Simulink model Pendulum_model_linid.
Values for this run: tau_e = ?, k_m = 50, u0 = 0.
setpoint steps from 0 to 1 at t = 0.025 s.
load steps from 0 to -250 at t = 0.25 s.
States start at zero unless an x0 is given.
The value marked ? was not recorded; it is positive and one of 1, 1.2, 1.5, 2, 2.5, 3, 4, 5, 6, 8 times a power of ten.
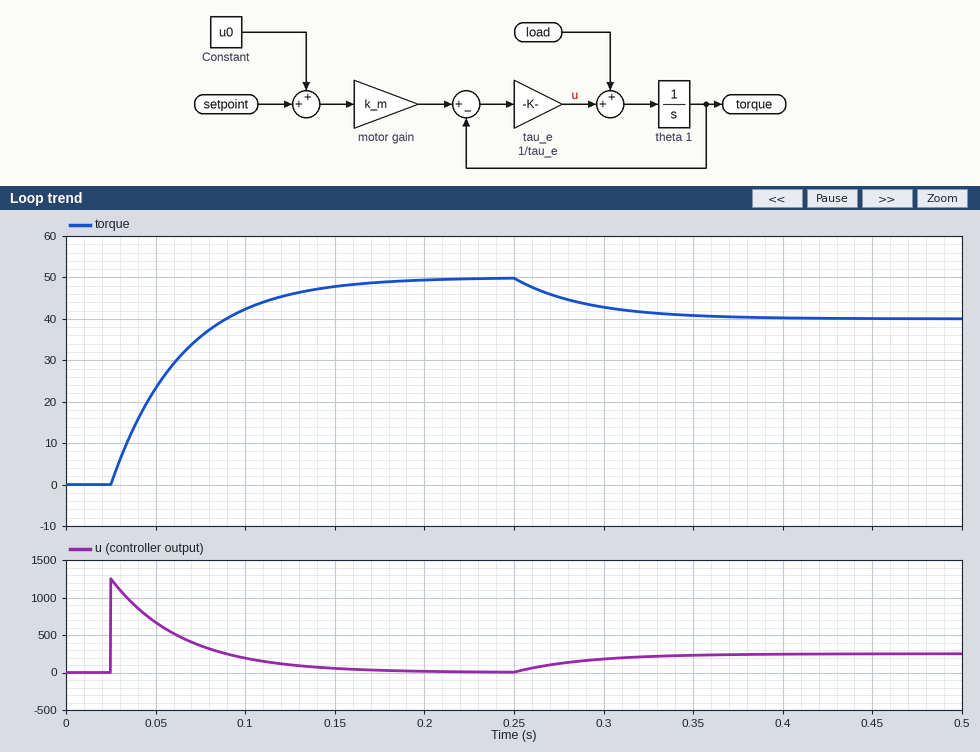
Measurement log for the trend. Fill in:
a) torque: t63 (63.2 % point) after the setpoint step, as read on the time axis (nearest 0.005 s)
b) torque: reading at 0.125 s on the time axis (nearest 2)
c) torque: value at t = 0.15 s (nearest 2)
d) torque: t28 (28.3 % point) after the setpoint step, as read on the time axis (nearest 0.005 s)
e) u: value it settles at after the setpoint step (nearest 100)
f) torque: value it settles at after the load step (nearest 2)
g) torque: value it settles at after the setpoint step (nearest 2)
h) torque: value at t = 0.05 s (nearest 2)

0.065 s
46
48
0.040 s
0
40
50
24
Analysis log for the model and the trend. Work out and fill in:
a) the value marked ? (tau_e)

0.04
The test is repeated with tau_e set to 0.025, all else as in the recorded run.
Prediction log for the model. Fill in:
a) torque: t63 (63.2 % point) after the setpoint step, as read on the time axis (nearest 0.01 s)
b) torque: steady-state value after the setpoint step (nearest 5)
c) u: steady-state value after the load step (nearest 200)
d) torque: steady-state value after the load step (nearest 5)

0.05 s
50
200
45
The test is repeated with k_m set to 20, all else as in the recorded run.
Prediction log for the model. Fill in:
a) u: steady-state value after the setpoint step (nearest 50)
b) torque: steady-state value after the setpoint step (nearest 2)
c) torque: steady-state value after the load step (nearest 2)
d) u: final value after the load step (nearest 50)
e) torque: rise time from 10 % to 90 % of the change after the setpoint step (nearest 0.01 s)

0
20
10
250
0.09 s
